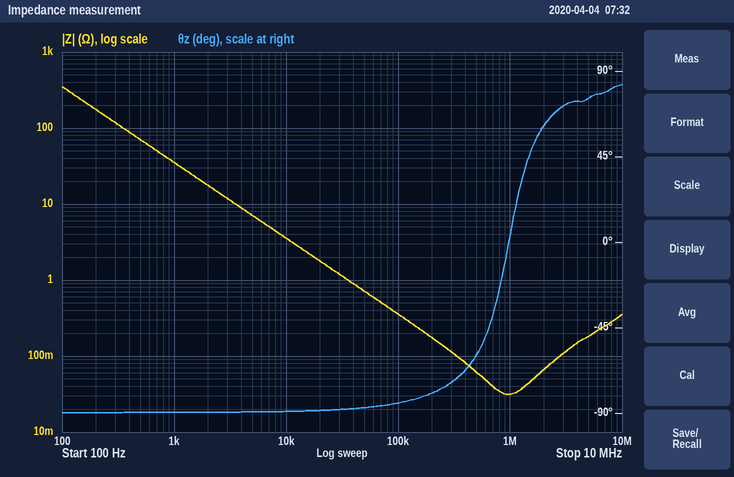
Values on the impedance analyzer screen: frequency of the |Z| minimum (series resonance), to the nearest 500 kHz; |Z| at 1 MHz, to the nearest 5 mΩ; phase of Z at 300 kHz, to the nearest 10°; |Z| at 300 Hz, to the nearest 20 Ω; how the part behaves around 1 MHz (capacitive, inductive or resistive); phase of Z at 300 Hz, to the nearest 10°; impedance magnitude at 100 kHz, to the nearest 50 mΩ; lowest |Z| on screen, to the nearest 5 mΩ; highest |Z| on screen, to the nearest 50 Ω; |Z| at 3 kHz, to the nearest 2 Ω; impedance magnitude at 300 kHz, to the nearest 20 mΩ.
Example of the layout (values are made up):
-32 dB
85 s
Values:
1.0 MHz
30 mΩ
-70°
120 Ω
resistive
-90°
350 mΩ
30 mΩ
350 Ω
12 Ω
120 mΩ
